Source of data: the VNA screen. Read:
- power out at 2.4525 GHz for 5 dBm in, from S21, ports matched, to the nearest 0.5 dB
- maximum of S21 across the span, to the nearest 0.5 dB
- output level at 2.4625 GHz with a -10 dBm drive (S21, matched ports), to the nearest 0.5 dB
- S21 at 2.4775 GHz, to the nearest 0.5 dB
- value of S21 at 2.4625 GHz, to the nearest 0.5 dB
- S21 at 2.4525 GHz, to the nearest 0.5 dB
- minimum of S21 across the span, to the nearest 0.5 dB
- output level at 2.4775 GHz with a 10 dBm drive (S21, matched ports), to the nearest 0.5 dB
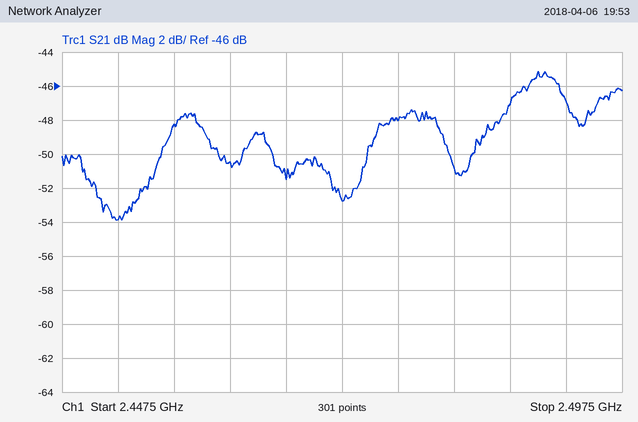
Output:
-49.0 dBm
-45.0 dB
-60.5 dBm
-48.0 dB
-50.5 dB
-54.0 dB
-54.0 dB
-38.0 dBm
